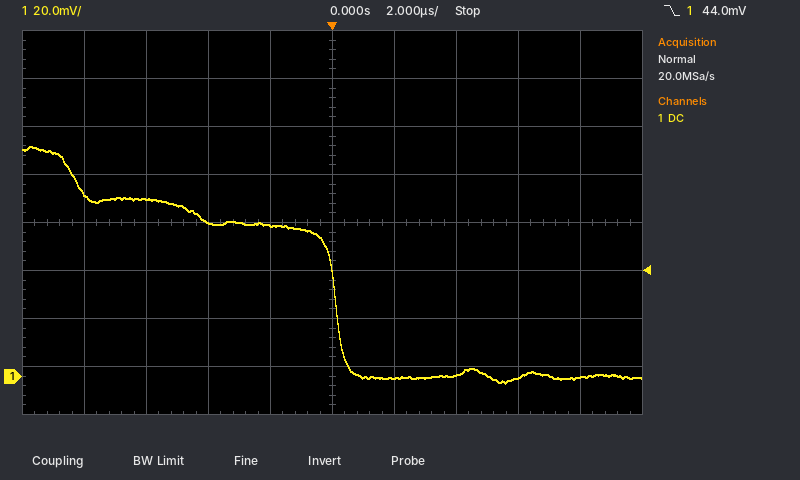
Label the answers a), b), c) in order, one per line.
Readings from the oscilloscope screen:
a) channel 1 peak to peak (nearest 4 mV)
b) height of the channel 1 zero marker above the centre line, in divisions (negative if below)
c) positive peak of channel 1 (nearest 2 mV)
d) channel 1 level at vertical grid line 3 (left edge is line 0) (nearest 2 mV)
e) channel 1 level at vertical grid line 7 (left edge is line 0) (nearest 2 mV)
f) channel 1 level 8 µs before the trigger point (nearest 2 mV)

a) 100 mV
b) -3.2 div
c) 96 mV
d) 64 mV
e) 0 mV
f) 76 mV
